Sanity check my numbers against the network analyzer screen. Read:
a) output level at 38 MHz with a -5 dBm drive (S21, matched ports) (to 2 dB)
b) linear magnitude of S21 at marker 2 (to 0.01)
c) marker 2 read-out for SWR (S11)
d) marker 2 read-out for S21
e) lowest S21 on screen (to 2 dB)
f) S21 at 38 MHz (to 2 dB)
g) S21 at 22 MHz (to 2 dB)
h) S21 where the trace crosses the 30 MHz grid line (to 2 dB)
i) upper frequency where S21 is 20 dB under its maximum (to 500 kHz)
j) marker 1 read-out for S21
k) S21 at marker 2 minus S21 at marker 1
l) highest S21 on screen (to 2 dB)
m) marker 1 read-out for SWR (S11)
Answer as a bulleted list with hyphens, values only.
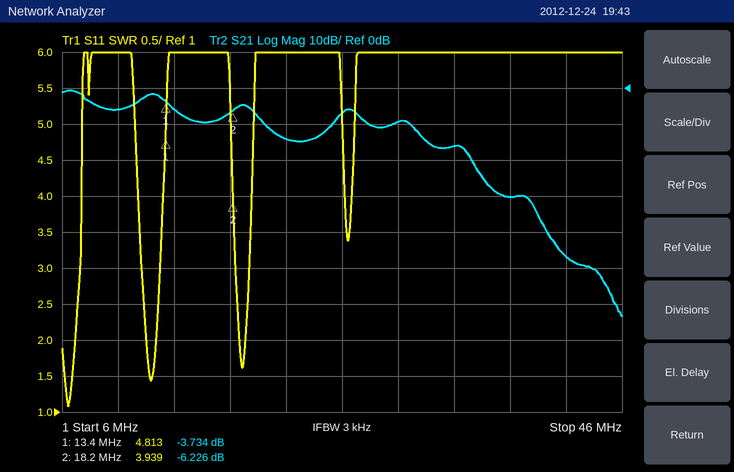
- -36 dBm
- 0.49
- 3.939
- -6.226 dB
- -64 dB
- -30 dB
- -14 dB
- -10 dB
- 35.5 MHz
- -3.734 dB
- -2.492 dB
- 0 dB
- 4.813
